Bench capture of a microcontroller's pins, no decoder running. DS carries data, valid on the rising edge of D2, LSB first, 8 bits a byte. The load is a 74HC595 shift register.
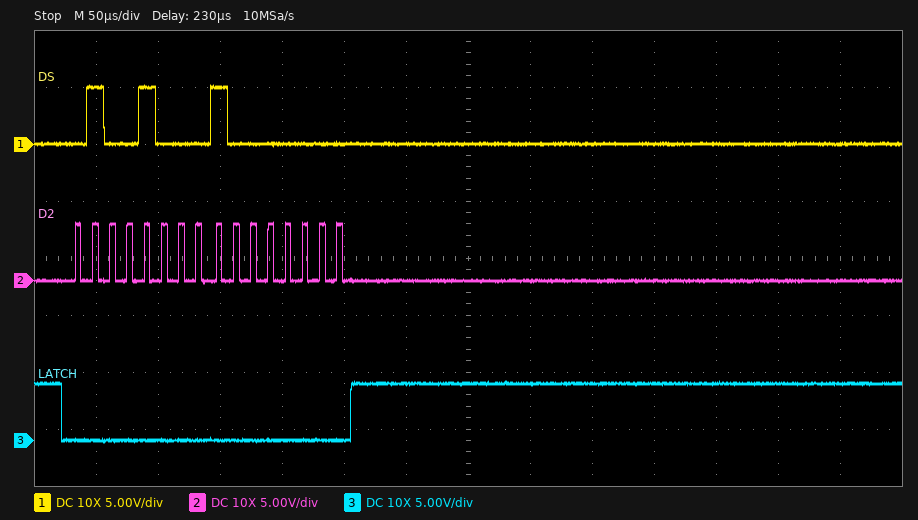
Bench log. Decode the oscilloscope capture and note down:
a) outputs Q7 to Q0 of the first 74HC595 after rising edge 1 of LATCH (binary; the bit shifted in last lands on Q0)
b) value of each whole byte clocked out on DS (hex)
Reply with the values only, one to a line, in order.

10000000
12 01
